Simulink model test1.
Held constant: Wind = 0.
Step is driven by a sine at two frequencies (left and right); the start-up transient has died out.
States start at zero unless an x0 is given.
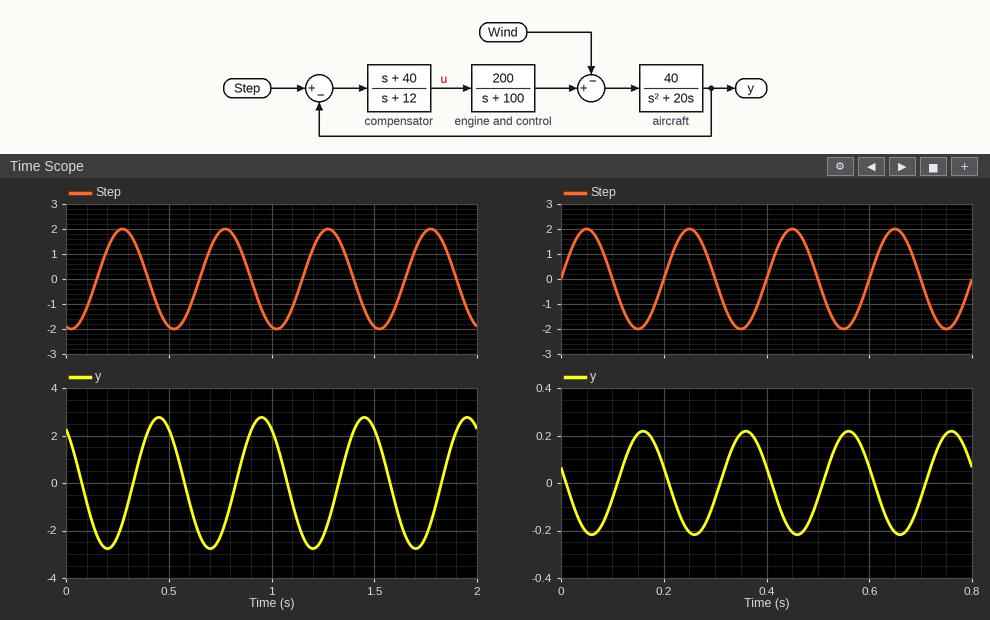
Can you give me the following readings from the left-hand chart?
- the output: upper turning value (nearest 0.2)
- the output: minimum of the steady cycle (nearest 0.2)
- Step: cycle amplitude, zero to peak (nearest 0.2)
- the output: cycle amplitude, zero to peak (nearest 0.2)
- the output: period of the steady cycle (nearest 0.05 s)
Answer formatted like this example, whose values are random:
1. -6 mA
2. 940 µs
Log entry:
1. 2.8
2. -2.8
3. 2.0
4. 2.8
5. 0.50 s
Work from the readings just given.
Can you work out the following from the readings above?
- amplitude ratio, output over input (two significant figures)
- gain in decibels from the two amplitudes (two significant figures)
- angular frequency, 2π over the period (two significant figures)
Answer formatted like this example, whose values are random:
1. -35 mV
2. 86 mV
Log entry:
1. 1.4
2. 2.9 dB
3. 13 rad/s
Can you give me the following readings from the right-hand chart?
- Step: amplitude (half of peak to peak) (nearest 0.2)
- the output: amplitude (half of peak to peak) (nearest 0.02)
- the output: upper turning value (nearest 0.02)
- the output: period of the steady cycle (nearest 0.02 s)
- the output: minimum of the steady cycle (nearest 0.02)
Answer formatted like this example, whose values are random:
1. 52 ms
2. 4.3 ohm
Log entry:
1. 2.0
2. 0.22
3. 0.22
4. 0.20 s
5. -0.22
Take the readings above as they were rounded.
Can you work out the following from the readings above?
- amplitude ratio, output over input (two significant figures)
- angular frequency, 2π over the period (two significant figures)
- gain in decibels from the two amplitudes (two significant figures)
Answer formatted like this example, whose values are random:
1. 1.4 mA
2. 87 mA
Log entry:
1. 0.11
2. 31 rad/s
3. -19 dB
